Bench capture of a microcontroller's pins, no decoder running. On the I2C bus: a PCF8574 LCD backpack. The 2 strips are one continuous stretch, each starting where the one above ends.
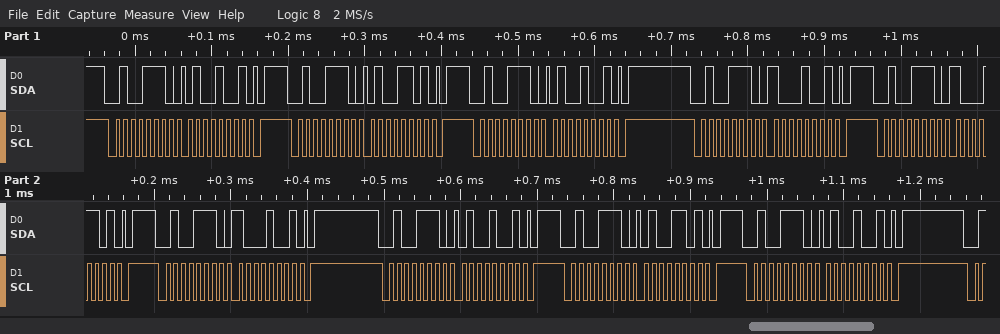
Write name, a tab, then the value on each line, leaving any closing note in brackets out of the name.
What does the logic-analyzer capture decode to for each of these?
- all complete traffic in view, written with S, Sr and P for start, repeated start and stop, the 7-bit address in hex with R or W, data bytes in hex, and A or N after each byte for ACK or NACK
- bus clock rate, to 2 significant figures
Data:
all complete traffic in view, written with S, Sr and P for start, repeated start and stop, the 7-bit address in hex with R or W, data bytes in hex, and A or N after each byte for ACK or NACK	S 27W A 49 A P S 27W A 4D A P S 27W A 49 A P S 27W A 89 A P S 27W A 8D A P S 27W A 89 A P S 27W A 49 A P S 27W A 4D A P S 27W A 49 A P
bus clock rate, to 2 significant figures	100 kHz
